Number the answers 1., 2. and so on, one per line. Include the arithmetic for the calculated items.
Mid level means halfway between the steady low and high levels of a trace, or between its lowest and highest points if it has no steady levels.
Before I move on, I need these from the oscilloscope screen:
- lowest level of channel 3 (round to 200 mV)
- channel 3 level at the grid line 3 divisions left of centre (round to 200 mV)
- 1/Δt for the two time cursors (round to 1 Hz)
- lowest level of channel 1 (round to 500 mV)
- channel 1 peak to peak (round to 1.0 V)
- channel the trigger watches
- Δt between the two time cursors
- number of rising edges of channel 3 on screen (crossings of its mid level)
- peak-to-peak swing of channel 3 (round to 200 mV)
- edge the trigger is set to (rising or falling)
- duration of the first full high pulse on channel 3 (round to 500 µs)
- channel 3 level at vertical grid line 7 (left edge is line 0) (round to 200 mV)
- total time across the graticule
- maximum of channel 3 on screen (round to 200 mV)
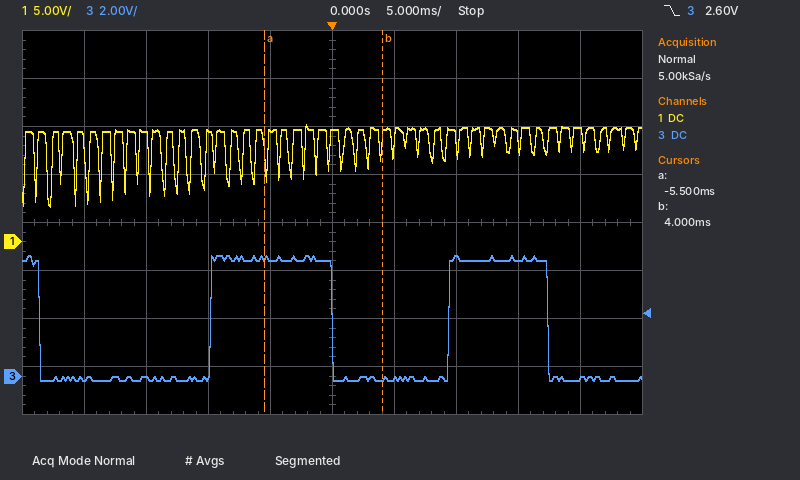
1. -200 mV
2. 0.0 V
3. 1 / 9.5 ms ≈ 105 Hz
4. 3.5 V
5. 9.0 V
6. channel 3
7. 4 ms − (-5.5 ms) = 9.5 ms
8. 2
9. 5.0 V − (-200 mV) = 5.2 V
10. falling
11. 10.0 ms
12. 5.0 V
13. 50 ms
14. 5.0 V
